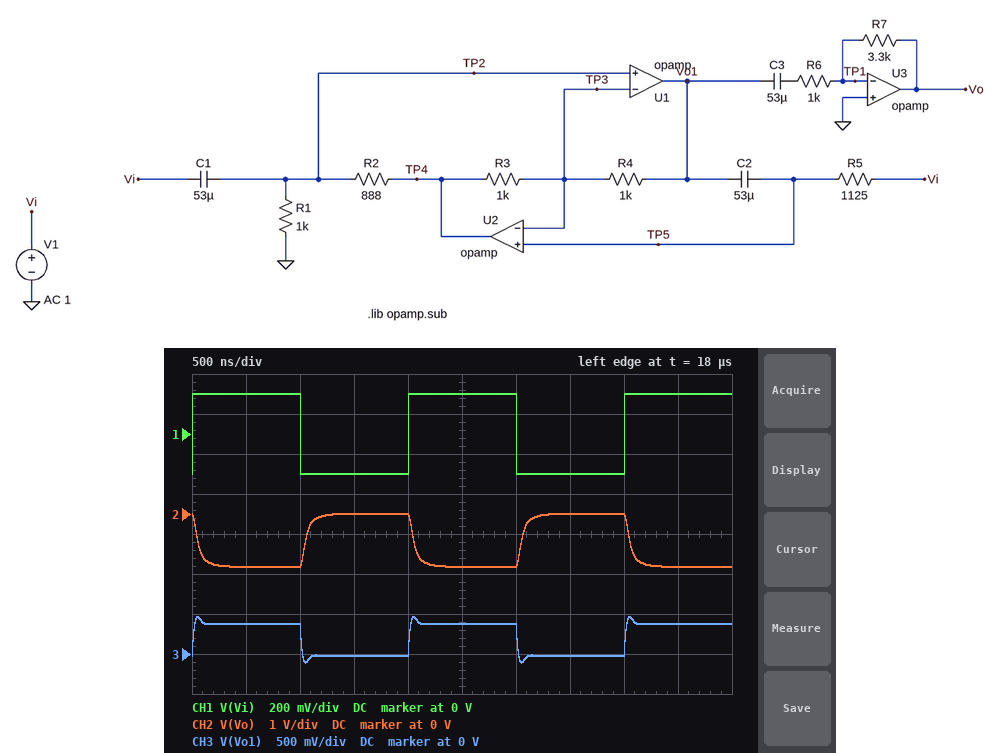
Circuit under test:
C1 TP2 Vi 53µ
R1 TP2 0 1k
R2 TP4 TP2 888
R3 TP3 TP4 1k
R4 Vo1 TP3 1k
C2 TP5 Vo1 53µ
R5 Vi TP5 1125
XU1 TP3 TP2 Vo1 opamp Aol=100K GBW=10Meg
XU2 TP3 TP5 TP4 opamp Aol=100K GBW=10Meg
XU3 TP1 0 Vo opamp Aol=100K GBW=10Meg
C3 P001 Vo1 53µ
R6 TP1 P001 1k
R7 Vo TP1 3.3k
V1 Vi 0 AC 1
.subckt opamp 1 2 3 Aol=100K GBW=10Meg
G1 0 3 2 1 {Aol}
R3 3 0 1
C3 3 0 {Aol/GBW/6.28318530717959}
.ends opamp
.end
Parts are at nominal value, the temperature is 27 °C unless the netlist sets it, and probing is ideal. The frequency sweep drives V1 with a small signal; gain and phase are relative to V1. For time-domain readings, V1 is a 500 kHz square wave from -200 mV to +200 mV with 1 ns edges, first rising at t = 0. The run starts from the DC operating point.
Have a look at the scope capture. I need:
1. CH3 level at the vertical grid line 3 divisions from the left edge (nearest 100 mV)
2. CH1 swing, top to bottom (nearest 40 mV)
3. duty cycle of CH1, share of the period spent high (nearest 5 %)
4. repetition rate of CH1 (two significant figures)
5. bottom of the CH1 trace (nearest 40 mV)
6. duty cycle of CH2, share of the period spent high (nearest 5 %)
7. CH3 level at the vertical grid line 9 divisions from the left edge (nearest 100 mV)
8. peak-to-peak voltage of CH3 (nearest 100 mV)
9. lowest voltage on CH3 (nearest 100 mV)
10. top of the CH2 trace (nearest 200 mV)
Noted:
0 V
400 mV
50 %
500 kHz
-200 mV
50 %
400 mV
600 mV
-100 mV
0 V
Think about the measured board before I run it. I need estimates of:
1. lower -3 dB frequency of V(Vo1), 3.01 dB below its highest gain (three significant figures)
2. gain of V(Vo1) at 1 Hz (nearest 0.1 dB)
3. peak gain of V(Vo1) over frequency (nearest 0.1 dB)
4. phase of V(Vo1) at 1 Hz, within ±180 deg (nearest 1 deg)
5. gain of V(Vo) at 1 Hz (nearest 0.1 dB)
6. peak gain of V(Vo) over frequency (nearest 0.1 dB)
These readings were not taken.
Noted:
2.74 Hz
-57.9 dB
0.8 dB
-20 deg
-57.5 dB
10.4 dB
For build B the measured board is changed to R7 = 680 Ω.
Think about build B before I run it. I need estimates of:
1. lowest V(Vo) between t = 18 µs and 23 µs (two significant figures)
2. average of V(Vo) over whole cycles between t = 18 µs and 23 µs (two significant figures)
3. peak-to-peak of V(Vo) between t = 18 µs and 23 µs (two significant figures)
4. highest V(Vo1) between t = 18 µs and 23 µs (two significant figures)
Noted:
-290 mV
-140 mV
310 mV
460 mV
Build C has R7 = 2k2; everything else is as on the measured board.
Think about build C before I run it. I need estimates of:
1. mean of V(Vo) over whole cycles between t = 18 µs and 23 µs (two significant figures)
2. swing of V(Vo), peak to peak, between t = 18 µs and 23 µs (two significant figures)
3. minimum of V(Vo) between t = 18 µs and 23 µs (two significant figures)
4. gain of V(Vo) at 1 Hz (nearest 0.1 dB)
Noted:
-440 mV
880 mV
-880 mV
-61.0 dB
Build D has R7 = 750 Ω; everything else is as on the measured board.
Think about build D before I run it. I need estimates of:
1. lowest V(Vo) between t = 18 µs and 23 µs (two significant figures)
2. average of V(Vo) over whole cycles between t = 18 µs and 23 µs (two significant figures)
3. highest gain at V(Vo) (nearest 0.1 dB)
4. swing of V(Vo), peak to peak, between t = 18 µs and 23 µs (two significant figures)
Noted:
-320 mV
-150 mV
-2.5 dB
340 mV
